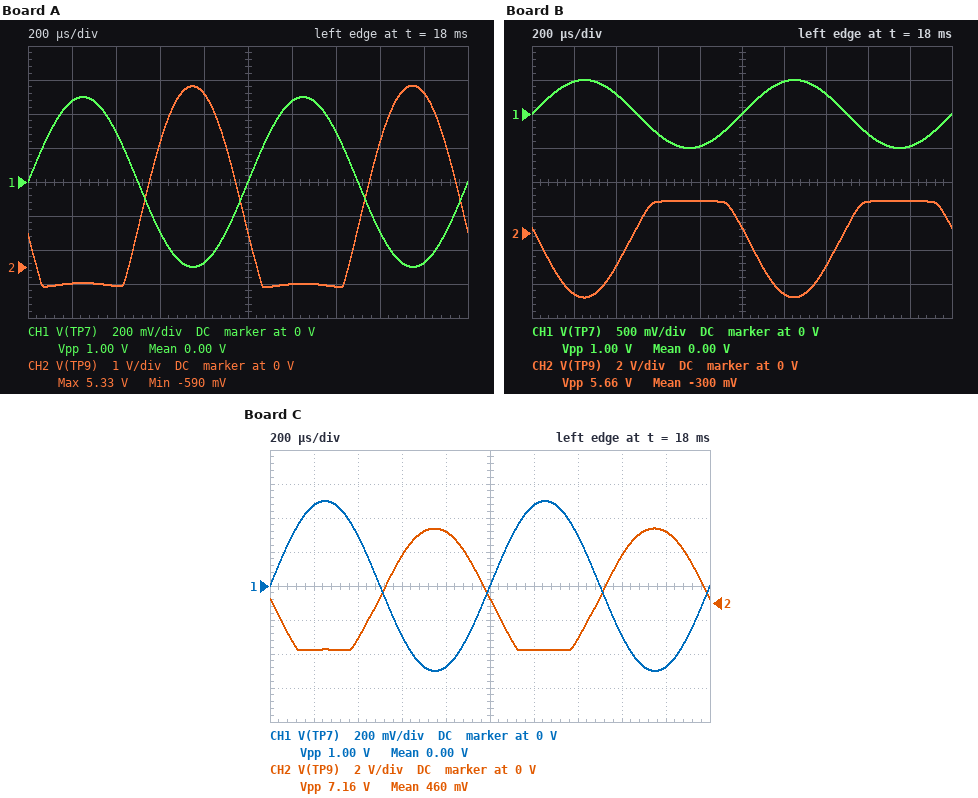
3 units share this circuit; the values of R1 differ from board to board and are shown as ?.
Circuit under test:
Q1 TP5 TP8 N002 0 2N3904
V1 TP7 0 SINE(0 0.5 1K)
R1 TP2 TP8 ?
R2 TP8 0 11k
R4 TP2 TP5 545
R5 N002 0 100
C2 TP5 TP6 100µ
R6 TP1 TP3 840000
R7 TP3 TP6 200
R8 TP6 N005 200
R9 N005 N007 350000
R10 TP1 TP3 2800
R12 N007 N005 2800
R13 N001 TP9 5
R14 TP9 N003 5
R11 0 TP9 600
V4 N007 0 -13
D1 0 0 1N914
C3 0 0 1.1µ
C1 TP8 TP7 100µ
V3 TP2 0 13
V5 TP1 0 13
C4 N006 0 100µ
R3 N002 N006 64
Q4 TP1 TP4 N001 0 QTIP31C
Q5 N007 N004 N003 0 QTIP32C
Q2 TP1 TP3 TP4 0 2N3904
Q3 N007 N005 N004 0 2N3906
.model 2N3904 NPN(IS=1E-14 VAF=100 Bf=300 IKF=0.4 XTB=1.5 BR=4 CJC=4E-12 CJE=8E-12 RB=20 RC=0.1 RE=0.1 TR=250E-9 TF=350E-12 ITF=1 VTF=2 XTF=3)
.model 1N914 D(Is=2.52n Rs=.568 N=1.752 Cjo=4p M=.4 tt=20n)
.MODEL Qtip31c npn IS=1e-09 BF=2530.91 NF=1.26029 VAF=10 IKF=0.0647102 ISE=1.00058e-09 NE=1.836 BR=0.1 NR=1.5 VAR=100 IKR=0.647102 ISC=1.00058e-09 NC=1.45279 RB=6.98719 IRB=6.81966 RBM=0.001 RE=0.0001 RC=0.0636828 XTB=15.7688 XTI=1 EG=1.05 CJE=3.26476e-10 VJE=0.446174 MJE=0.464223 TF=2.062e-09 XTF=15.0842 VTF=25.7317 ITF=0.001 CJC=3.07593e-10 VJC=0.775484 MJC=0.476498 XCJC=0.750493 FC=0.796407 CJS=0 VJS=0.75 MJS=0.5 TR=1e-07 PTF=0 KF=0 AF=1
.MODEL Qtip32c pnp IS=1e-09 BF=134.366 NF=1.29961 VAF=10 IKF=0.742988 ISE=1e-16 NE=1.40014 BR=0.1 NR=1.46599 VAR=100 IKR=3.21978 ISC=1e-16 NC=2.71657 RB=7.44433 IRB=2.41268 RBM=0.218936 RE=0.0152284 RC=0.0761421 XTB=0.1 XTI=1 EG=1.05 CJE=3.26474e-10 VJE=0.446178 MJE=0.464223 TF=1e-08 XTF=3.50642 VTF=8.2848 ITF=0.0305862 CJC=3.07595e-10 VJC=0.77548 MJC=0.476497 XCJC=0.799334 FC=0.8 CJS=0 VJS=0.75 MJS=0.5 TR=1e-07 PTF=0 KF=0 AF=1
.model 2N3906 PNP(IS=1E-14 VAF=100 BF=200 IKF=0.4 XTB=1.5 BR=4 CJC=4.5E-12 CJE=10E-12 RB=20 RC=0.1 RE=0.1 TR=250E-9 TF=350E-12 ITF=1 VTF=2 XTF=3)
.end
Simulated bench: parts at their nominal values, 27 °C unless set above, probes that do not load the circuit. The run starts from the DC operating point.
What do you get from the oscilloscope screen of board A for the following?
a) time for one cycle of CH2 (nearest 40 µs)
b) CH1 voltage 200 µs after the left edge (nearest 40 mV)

1.00 ms
480 mV
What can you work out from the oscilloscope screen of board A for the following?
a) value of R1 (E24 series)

33 kΩ
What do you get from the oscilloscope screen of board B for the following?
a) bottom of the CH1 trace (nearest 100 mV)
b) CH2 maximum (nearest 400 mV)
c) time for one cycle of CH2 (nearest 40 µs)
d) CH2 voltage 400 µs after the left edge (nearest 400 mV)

-500 mV
2.0 V
1.00 ms
-2.0 V
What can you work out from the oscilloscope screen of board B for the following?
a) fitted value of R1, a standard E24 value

91 kΩ
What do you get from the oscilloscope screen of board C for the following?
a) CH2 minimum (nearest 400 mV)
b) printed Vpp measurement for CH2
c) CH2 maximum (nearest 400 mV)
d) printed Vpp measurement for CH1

-2.8 V
7.16 V
4.4 V
1.00 V
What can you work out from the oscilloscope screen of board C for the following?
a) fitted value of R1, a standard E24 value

43 kΩ
